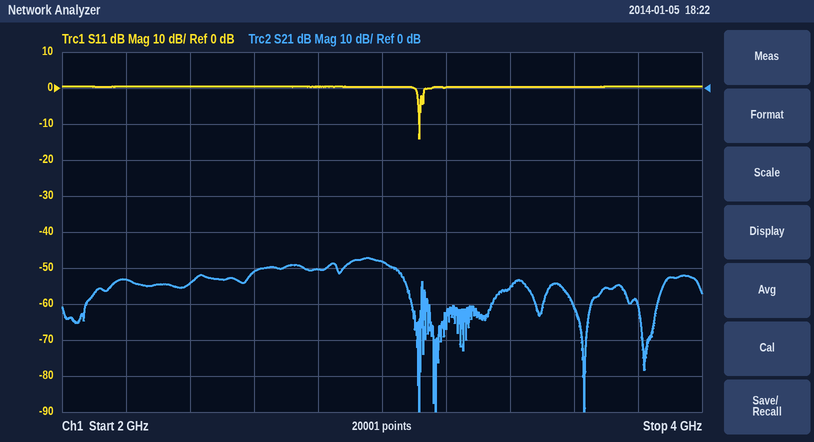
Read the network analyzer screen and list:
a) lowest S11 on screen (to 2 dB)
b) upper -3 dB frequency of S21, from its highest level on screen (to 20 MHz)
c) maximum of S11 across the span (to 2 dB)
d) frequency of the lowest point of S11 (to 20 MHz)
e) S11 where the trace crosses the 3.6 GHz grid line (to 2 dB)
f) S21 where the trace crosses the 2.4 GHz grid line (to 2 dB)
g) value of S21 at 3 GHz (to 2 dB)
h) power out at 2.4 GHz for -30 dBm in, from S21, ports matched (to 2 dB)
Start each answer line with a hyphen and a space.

- -14 dB
- 3.04 GHz
- 0 dB
- 3.12 GHz
- 0 dB
- -54 dB
- -48 dB
- -84 dBm
